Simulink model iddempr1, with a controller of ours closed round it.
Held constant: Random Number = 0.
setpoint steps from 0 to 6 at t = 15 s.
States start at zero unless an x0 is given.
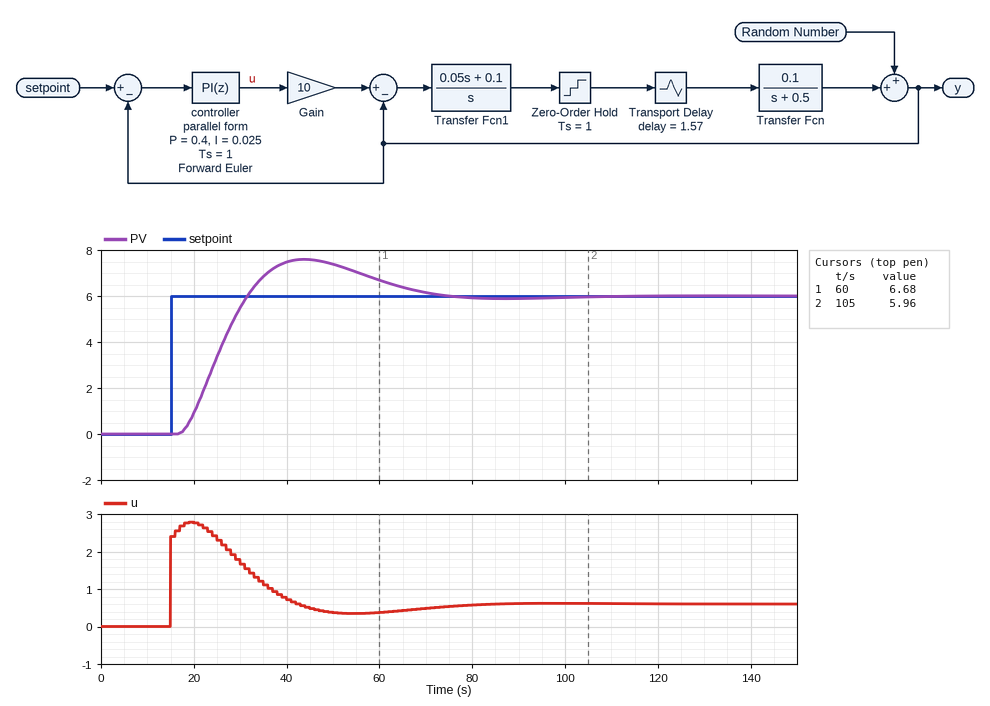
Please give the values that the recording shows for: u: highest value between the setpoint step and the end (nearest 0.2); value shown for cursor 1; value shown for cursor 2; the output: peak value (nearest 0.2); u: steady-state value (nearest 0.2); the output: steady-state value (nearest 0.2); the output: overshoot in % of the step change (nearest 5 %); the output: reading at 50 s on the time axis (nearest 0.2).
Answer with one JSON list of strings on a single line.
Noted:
["2.8", "6.68", "5.96", "7.6", "0.6", "6.0", "25 %", "7.4"]
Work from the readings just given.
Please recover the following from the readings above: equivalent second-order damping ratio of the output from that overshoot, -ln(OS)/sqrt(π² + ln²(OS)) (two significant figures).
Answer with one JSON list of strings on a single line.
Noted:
["0.40"]
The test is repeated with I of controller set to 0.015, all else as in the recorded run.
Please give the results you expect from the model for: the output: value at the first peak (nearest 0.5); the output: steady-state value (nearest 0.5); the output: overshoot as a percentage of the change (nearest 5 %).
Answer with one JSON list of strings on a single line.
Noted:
["6.5", "6.0", "10 %"]
